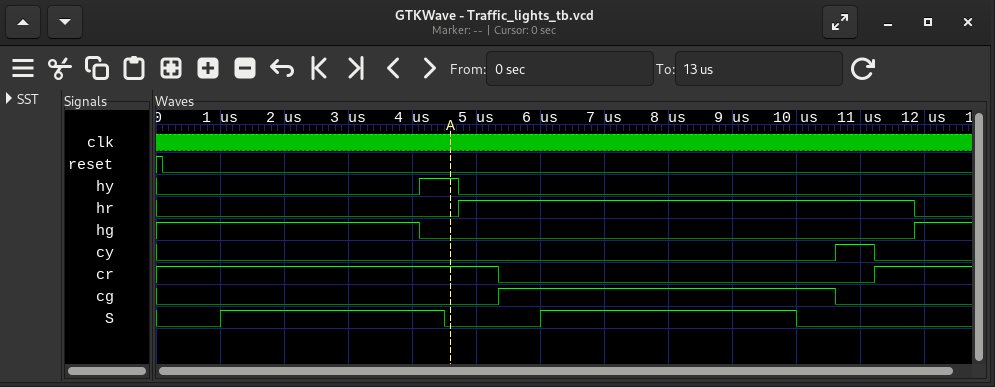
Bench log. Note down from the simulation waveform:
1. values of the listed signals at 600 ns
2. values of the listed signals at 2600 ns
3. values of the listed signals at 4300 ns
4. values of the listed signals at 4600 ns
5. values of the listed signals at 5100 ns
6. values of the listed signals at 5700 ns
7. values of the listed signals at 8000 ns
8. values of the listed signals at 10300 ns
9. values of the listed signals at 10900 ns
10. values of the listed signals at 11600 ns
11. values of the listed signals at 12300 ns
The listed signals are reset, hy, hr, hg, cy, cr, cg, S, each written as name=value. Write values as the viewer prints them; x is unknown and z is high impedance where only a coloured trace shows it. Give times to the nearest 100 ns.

reset=0, hy=0, hr=0, hg=1, cy=0, cr=1, cg=0, S=0
reset=0, hy=0, hr=0, hg=1, cy=0, cr=1, cg=0, S=1
reset=0, hy=1, hr=0, hg=0, cy=0, cr=1, cg=0, S=1
reset=0, hy=1, hr=0, hg=0, cy=0, cr=1, cg=0, S=0
reset=0, hy=0, hr=1, hg=0, cy=0, cr=1, cg=0, S=0
reset=0, hy=0, hr=1, hg=0, cy=0, cr=0, cg=1, S=0
reset=0, hy=0, hr=1, hg=0, cy=0, cr=0, cg=1, S=1
reset=0, hy=0, hr=1, hg=0, cy=0, cr=0, cg=1, S=0
reset=0, hy=0, hr=1, hg=0, cy=1, cr=0, cg=0, S=0
reset=0, hy=0, hr=1, hg=0, cy=0, cr=1, cg=0, S=0
reset=0, hy=0, hr=0, hg=1, cy=0, cr=1, cg=0, S=0
